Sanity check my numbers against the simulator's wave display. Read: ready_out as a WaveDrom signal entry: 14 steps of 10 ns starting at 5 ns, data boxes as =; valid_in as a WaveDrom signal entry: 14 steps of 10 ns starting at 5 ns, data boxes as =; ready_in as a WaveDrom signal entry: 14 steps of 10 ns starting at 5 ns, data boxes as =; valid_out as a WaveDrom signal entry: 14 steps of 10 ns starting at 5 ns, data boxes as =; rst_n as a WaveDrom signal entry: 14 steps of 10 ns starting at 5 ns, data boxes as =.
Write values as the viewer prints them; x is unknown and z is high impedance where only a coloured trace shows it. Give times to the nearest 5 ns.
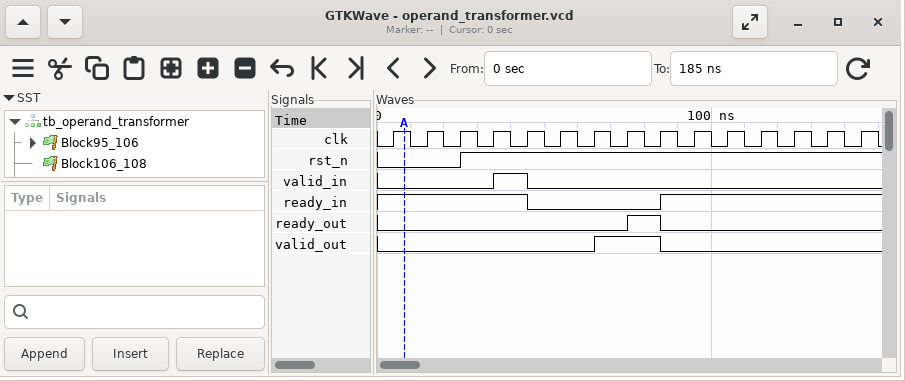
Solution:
{name: 'ready_out', wave: '0......10.....'}
{name: 'valid_in', wave: '0..10.........'}
{name: 'ready_in', wave: '1...0...1.....'}
{name: 'valid_out', wave: '0.....1.0.....'}
{name: 'rst_n', wave: '0.1...........'}
